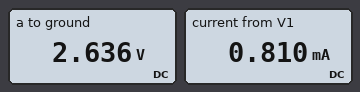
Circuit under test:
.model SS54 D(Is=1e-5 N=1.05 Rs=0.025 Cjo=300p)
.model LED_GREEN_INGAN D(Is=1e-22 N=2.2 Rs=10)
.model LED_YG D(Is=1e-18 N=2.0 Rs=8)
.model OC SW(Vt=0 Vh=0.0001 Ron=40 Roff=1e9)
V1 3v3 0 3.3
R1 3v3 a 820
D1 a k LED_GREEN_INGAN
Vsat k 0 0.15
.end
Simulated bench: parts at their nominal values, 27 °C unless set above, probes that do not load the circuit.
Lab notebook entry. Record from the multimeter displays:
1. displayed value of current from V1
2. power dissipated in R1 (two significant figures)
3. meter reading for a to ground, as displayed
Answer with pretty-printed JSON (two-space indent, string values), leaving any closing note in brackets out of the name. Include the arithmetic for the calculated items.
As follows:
{
  "displayed value of current from V1": "0.810 mA",
  "power dissipated in R1": "(3.3 V - 2.636 V)^2 / 820 Ω = 540 µW",
  "meter reading for a to ground, as displayed": "2.636 V"
}
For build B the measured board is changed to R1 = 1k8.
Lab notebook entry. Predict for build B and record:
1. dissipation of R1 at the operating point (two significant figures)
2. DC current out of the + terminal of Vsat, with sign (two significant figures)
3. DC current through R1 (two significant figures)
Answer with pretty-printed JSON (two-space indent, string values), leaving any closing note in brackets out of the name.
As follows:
{
  "dissipation of R1 at the operating point": "280 µW",
  "DC current out of the + terminal of Vsat, with sign": "-390 µA",
  "DC current through R1": "390 µA"
}
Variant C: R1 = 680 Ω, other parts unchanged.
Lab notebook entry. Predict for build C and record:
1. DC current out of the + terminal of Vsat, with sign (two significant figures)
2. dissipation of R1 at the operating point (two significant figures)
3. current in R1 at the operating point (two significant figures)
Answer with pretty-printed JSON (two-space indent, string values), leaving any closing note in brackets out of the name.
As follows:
{
  "DC current out of the + terminal of Vsat, with sign": "-960 µA",
  "dissipation of R1 at the operating point": "630 µW",
  "current in R1 at the operating point": "960 µA"
}
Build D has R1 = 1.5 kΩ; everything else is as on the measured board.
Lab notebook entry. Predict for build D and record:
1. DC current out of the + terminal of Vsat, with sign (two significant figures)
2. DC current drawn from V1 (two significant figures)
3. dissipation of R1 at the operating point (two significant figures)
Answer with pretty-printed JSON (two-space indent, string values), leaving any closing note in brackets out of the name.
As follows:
{
  "DC current out of the + terminal of Vsat, with sign": "-470 µA",
  "DC current drawn from V1": "470 µA",
  "dissipation of R1 at the operating point": "330 µW"
}
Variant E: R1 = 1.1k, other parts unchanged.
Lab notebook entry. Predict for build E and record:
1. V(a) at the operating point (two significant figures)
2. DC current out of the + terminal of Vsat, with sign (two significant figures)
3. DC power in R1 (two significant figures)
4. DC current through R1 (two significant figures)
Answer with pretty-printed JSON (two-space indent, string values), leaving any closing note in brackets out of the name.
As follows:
{
  "V(a) at the operating point": "2.6 V",
  "DC current out of the + terminal of Vsat, with sign": "-620 µA",
  "DC power in R1": "420 µW",
  "DC current through R1": "620 µA"
}
